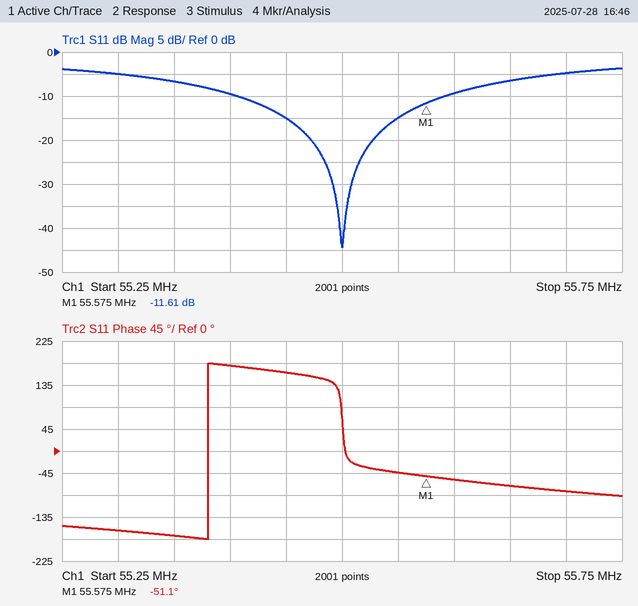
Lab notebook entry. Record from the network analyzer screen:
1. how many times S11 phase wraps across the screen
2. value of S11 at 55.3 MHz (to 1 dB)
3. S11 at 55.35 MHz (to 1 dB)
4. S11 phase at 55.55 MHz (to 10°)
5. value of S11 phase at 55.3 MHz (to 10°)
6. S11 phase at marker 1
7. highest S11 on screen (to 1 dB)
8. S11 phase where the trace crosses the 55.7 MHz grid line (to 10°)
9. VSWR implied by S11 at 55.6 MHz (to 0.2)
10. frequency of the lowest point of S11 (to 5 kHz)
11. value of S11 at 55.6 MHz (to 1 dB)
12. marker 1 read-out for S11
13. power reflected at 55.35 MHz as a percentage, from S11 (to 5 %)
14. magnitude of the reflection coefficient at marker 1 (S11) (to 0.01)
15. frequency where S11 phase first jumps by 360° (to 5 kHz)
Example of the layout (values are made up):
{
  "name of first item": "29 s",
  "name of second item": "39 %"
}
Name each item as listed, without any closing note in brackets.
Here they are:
{
  "how many times S11 phase wraps across the screen": "1",
  "value of S11 at 55.3 MHz": "-5 dB",
  "S11 at 55.35 MHz": "-7 dB",
  "S11 phase at 55.55 MHz": "-40°",
  "value of S11 phase at 55.3 MHz": "-160°",
  "S11 phase at marker 1": "-51.1°",
  "highest S11 on screen": "-4 dB",
  "S11 phase where the trace crosses the 55.7 MHz grid line": "-80°",
  "VSWR implied by S11 at 55.6 MHz": "2.0",
  "frequency of the lowest point of S11": "55.500 MHz",
  "value of S11 at 55.6 MHz": "-9 dB",
  "marker 1 read-out for S11": "-11.61 dB",
  "power reflected at 55.35 MHz as a percentage, from S11": "20 %",
  "magnitude of the reflection coefficient at marker 1 (S11)": "0.26",
  "frequency where S11 phase first jumps by 360°": "55.380 MHz"
}
